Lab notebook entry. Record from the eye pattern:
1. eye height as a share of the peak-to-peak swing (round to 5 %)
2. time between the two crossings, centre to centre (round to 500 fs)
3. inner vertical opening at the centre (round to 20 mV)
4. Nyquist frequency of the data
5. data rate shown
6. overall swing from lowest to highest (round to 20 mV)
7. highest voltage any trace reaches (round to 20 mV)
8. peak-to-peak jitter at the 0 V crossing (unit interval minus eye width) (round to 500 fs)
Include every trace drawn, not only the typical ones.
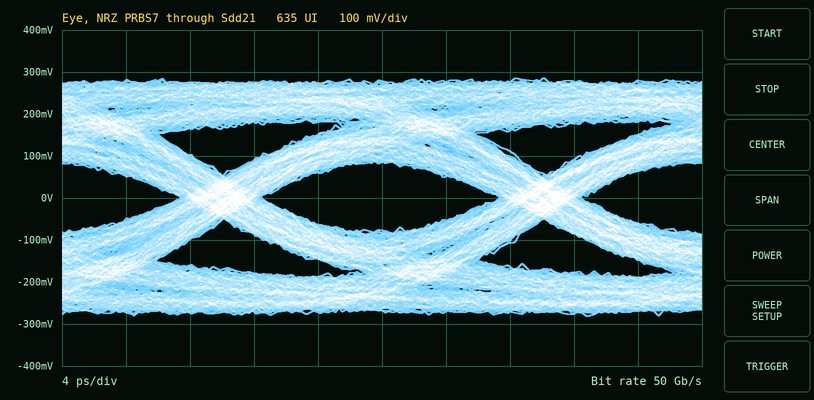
30 %
20.0 ps
160 mV
25 GHz
50 Gb/s
560 mV
280 mV
5.0 ps
